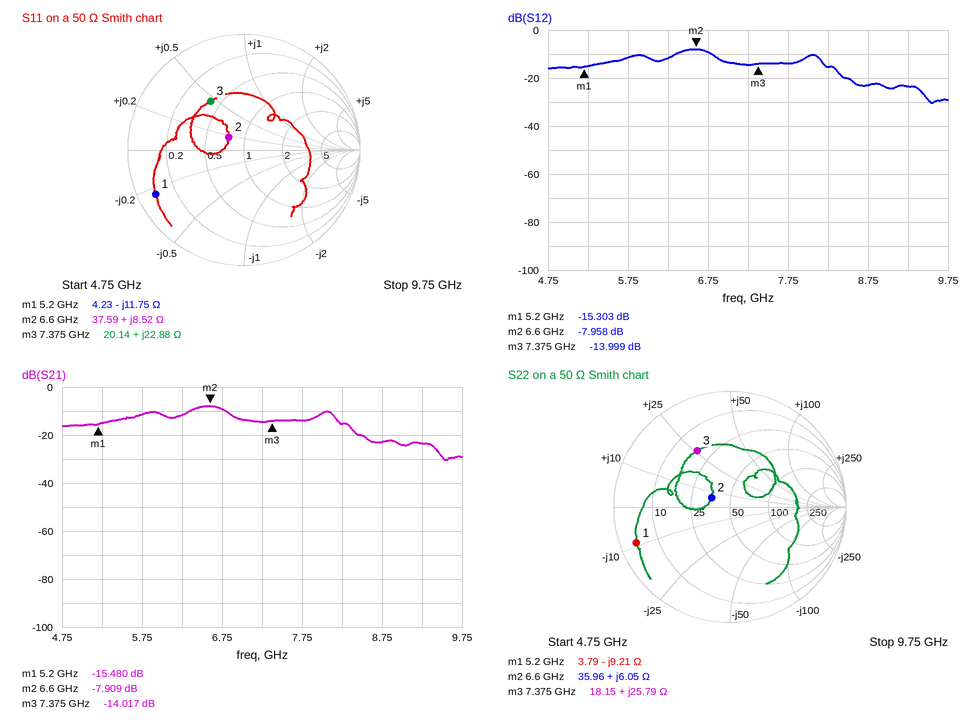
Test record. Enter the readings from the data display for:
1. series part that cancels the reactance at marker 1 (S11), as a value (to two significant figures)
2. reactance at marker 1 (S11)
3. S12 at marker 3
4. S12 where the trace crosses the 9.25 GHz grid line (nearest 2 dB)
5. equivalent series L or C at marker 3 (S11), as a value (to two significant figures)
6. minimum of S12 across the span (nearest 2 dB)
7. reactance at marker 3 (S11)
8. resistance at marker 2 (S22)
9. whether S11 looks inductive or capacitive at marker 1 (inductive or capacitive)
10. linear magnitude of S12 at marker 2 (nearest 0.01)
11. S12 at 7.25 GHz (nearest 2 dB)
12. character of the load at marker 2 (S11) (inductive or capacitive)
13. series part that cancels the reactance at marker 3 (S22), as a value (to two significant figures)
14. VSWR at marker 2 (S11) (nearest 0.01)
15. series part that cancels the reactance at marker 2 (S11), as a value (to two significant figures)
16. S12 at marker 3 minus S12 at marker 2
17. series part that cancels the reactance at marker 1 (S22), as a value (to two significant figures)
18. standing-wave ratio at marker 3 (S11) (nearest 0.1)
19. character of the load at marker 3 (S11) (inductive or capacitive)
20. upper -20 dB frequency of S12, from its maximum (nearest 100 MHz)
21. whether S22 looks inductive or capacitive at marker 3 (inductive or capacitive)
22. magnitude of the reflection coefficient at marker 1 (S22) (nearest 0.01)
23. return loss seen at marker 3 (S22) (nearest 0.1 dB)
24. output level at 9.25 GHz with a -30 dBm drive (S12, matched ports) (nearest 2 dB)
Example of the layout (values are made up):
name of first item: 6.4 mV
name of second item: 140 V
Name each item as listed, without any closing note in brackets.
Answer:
series part that cancels the reactance at marker 1 (S11), as a value: 360 pH
reactance at marker 1: -11.75 Ω
S12 at marker 3: -13.999 dB
S12 where the trace crosses the 9.25 GHz grid line: -24 dB
equivalent series L or C at marker 3 (S11), as a value: 490 pH
minimum of S12 across the span: -30 dB
reactance at marker 3: +22.88 Ω
resistance at marker 2: 35.96 Ω
whether S11 looks inductive or capacitive at marker 1: capacitive
linear magnitude of S12 at marker 2: 0.40
S12 at 7.25 GHz: -14 dB
character of the load at marker 2 (S11): inductive
series part that cancels the reactance at marker 3 (S22), as a value: 840 fF
VSWR at marker 2 (S11): 1.41
series part that cancels the reactance at marker 2 (S11), as a value: 2.8 pF
S12 at marker 3 minus S12 at marker 2: -6.041 dB
series part that cancels the reactance at marker 1 (S22), as a value: 280 pH
standing-wave ratio at marker 3 (S11): 3.1
character of the load at marker 3 (S11): inductive
upper -20 dB frequency of S12, from its maximum: 9.5 GHz
whether S22 looks inductive or capacitive at marker 3: inductive
magnitude of the reflection coefficient at marker 1 (S22): 0.86
return loss seen at marker 3 (S22): 5.0 dB
output level at 9.25 GHz with a -30 dBm drive (S12, matched ports): -54 dBm
